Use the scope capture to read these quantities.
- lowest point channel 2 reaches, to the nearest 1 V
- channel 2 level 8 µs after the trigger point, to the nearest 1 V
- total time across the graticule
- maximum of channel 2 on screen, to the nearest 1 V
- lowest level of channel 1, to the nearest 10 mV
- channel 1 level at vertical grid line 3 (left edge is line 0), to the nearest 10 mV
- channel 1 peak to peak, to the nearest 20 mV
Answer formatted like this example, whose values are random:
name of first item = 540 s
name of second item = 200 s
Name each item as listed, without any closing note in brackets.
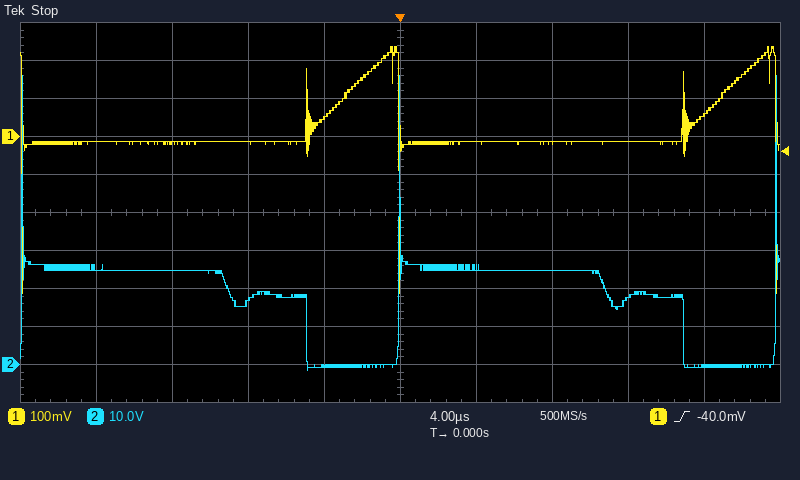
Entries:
lowest point channel 2 reaches, to the nearest 1 V = -2 V
channel 2 level 8 µs after the trigger point, to the nearest 1 V = 25 V
total time across the graticule = 40 µs
maximum of channel 2 on screen, to the nearest 1 V = 76 V
lowest level of channel 1, to the nearest 10 mV = -410 mV
channel 1 level at vertical grid line 3 (left edge is line 0), to the nearest 10 mV = -20 mV
channel 1 peak to peak, to the nearest 20 mV = 640 mV
